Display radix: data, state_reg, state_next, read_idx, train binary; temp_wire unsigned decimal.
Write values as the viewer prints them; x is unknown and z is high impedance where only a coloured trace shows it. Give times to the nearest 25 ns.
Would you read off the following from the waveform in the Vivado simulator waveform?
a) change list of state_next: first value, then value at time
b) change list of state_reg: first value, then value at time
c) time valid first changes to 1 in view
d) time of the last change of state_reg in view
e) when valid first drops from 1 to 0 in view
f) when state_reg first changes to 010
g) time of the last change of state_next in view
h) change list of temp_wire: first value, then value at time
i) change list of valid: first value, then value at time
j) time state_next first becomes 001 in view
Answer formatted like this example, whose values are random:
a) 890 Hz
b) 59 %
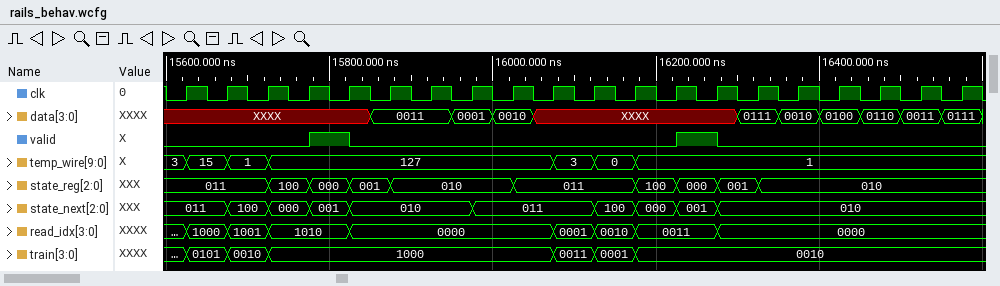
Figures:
a) 011, 100 at 15675 ns, 000 at 15725 ns, 001 at 15775 ns, 010 at 15825 ns, 011 at 15975 ns, 100 at 16125 ns, 000 at 16175 ns, 001 at 16225 ns, 010 at 16275 ns
b) 011, 100 at 15725 ns, 000 at 15775 ns, 001 at 15825 ns, 010 at 15875 ns, 011 at 16025 ns, 100 at 16175 ns, 000 at 16225 ns, 001 at 16275 ns, 010 at 16325 ns
c) 15775 ns
d) 16325 ns
e) 15825 ns
f) 15875 ns
g) 16275 ns
h) 3, 15 at 15625 ns, 1 at 15675 ns, 127 at 15725 ns, 3 at 16075 ns, 0 at 16125 ns, 1 at 16175 ns
i) 0, 1 at 15775 ns, 0 at 15825 ns, 1 at 16225 ns, 0 at 16275 ns
j) 15775 ns
